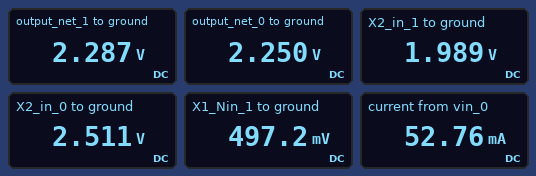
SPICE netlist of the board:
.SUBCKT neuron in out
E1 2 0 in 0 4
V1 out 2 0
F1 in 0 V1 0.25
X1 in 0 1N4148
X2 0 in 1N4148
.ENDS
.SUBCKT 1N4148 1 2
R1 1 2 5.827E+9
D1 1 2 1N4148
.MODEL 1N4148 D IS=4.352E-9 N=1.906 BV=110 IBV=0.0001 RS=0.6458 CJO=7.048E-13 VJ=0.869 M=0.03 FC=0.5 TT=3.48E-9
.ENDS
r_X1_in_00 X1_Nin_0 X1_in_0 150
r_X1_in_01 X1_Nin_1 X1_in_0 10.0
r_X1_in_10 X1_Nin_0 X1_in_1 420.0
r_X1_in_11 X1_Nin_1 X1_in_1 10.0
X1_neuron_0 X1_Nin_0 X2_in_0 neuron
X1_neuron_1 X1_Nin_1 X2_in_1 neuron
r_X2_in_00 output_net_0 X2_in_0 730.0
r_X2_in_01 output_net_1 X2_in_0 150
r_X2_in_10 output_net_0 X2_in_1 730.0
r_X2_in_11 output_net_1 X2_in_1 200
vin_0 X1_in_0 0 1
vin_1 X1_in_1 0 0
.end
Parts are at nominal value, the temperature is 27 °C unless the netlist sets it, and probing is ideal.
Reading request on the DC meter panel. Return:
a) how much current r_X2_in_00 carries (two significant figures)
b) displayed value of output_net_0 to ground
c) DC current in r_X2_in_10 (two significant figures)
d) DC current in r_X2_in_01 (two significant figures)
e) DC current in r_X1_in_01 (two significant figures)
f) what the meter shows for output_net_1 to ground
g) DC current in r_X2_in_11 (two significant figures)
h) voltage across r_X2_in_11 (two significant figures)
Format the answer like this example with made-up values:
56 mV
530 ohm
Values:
360 µA
2.250 V
360 µA
1.5 mA
50 mA
2.287 V
1.5 mA
300 mV
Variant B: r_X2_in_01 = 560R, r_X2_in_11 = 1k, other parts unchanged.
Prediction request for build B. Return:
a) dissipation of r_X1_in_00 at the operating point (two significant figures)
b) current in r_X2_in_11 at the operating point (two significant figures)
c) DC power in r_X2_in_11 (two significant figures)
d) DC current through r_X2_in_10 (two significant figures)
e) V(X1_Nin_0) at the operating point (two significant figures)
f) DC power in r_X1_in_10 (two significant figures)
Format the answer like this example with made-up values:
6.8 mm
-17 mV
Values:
970 µW
310 µA
96 µW
330 µA
620 mV
910 µW
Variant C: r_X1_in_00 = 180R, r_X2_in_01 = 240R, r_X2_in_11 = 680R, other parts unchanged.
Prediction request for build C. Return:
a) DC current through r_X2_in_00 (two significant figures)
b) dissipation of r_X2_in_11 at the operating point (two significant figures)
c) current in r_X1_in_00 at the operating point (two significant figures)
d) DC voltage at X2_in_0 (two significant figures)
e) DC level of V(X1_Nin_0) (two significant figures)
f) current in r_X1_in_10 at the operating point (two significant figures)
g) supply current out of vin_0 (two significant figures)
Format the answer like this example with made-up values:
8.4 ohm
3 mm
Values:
290 µA
150 µW
2.2 mA
2.4 V
610 mV
1.4 mA
52 mA
